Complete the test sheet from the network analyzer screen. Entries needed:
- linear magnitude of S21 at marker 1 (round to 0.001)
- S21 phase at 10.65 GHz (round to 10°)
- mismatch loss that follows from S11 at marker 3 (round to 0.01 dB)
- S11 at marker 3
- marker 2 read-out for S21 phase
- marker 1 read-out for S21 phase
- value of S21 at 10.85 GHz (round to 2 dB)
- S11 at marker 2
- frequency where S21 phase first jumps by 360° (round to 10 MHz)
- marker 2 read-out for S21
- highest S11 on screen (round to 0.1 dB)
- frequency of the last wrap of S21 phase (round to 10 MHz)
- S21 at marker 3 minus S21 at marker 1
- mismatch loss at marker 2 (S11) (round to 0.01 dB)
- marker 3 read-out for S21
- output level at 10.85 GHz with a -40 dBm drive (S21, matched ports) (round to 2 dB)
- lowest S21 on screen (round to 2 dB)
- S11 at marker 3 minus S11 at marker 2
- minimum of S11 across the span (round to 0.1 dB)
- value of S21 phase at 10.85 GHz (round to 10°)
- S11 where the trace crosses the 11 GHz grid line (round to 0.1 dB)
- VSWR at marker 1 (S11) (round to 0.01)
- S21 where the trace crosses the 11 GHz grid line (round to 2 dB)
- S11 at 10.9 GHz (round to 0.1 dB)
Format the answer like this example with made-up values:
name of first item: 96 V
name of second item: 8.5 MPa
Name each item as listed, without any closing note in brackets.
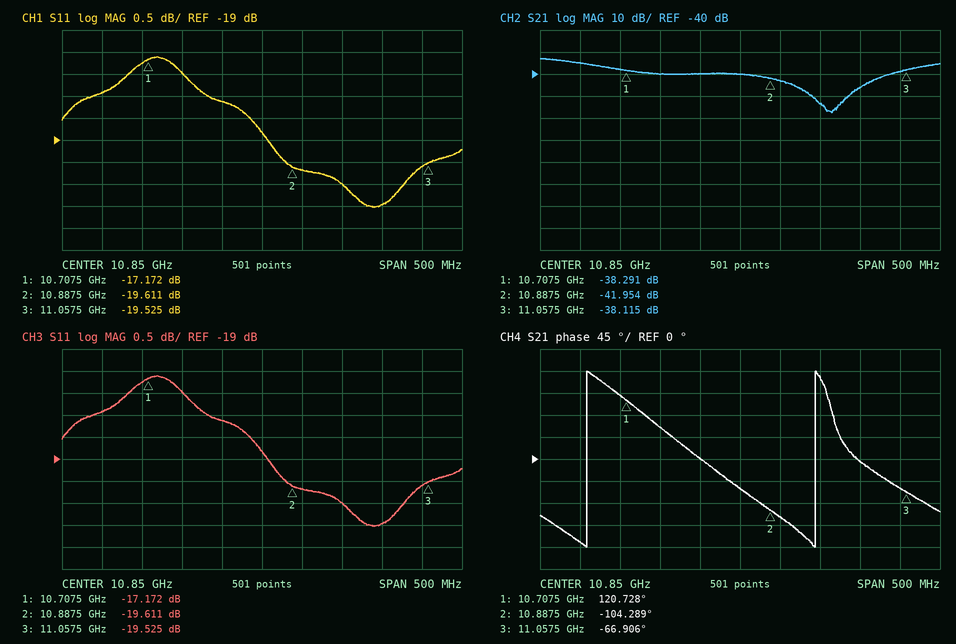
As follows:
linear magnitude of S21 at marker 1: 0.012
S21 phase at 10.65 GHz: -170°
mismatch loss that follows from S11 at marker 3: 0.05 dB
S11 at marker 3: -19.525 dB
marker 2 read-out for S21 phase: -104.289°
marker 1 read-out for S21 phase: 120.728°
value of S21 at 10.85 GHz: -40 dB
S11 at marker 2: -19.611 dB
frequency where S21 phase first jumps by 360°: 10.66 GHz
marker 2 read-out for S21: -41.954 dB
highest S11 on screen: -17.1 dB
frequency of the last wrap of S21 phase: 10.94 GHz
S21 at marker 3 minus S21 at marker 1: 0.176 dB
mismatch loss at marker 2 (S11): 0.05 dB
marker 3 read-out for S21: -38.115 dB
output level at 10.85 GHz with a -40 dBm drive (S21, matched ports): -80 dBm
lowest S21 on screen: -58 dB
S11 at marker 3 minus S11 at marker 2: 0.086 dB
minimum of S11 across the span: -20.5 dB
value of S21 phase at 10.85 GHz: -60°
S11 where the trace crosses the 11 GHz grid line: -20.5 dB
VSWR at marker 1 (S11): 1.32
S21 where the trace crosses the 11 GHz grid line: -46 dB
S11 at 10.9 GHz: -19.7 dB
